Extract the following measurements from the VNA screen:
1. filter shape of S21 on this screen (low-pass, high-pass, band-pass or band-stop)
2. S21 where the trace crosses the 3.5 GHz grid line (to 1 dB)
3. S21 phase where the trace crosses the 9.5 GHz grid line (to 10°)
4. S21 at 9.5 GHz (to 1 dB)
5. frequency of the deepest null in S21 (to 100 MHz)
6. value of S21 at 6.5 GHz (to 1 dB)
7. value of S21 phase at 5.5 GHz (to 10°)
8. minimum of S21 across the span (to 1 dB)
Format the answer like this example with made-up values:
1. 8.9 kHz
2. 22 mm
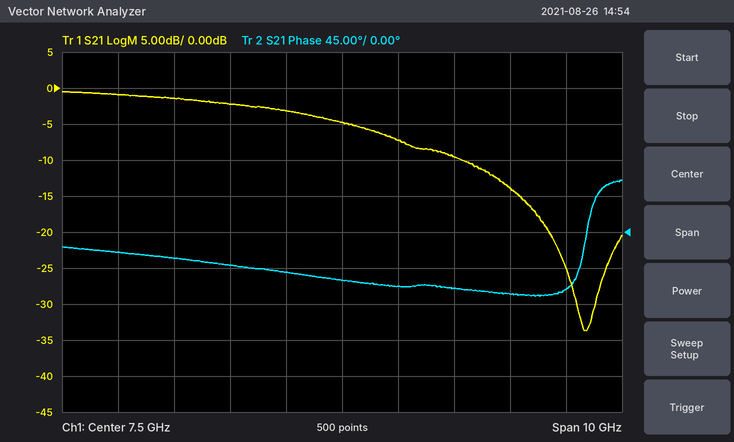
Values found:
1. low-pass
2. -1 dB
3. -70°
4. -10 dB
5. 11.8 GHz
6. -3 dB
7. -40°
8. -34 dB
